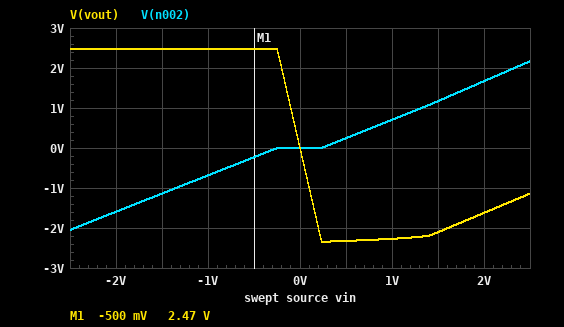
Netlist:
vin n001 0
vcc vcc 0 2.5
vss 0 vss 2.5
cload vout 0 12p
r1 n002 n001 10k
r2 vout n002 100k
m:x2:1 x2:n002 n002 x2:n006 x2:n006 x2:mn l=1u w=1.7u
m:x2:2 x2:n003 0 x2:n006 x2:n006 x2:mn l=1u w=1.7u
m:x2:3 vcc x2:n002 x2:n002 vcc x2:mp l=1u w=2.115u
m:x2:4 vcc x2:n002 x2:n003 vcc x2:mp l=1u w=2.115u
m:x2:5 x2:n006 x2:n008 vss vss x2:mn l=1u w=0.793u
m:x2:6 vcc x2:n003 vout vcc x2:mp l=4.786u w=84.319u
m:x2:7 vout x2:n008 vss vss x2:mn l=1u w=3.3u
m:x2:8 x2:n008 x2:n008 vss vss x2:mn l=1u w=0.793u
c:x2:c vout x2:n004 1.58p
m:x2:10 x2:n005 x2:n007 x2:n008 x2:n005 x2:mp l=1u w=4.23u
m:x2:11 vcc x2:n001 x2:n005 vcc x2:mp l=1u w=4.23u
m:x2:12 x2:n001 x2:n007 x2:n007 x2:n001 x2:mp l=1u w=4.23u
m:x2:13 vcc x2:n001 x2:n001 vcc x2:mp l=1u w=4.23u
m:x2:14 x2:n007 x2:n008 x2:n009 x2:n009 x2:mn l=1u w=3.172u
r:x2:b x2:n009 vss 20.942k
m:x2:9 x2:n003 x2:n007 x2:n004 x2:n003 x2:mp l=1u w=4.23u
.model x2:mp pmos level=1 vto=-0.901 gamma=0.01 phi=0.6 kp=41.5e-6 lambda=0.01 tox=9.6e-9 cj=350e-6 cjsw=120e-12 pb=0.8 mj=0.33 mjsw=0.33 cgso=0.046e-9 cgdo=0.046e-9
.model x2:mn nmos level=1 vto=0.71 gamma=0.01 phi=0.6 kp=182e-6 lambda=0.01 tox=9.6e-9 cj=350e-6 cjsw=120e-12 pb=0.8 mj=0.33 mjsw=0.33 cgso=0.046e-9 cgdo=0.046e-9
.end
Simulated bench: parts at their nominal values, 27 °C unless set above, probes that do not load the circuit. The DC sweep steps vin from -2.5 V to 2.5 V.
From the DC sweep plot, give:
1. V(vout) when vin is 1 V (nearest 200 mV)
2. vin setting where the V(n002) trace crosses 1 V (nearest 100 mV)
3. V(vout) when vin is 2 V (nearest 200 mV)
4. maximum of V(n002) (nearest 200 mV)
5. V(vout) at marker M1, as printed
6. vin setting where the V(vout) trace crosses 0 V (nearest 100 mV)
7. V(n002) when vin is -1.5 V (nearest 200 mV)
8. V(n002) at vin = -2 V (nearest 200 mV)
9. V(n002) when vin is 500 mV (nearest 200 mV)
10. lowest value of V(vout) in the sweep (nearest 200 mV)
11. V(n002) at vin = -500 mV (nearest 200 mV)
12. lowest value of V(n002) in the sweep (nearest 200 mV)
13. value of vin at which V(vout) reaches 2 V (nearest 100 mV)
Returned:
-2.2 V
1.3 V
-1.6 V
2.2 V
2.47 V
0 V
-1.2 V
-1.6 V
200 mV
-2.4 V
-200 mV
-2.0 V
-200 mV
